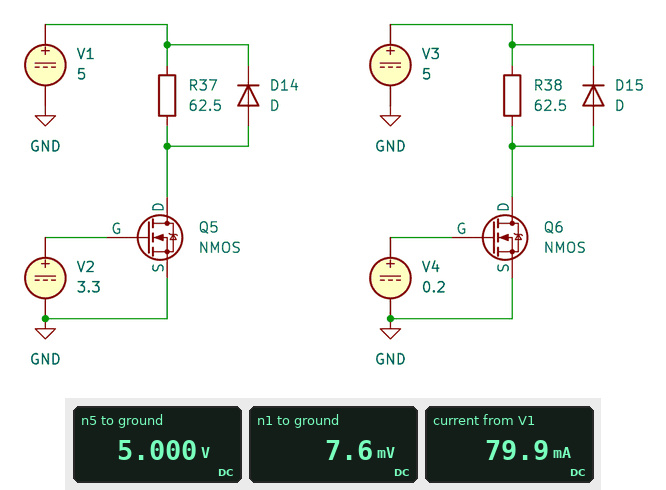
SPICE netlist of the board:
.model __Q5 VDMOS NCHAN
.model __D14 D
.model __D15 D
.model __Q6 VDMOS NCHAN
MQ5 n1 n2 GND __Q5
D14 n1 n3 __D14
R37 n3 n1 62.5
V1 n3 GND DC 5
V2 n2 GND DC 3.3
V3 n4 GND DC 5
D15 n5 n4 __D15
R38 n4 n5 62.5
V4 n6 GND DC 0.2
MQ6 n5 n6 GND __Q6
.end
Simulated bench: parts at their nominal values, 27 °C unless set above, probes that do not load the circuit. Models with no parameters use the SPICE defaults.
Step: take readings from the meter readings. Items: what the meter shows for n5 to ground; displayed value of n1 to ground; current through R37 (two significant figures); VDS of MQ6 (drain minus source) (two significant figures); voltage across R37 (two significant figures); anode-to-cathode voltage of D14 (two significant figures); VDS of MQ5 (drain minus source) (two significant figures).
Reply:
5.000 V
7.6 mV
80 mA
5.0 V
5.0 V
-5.0 V
7.6 mV
